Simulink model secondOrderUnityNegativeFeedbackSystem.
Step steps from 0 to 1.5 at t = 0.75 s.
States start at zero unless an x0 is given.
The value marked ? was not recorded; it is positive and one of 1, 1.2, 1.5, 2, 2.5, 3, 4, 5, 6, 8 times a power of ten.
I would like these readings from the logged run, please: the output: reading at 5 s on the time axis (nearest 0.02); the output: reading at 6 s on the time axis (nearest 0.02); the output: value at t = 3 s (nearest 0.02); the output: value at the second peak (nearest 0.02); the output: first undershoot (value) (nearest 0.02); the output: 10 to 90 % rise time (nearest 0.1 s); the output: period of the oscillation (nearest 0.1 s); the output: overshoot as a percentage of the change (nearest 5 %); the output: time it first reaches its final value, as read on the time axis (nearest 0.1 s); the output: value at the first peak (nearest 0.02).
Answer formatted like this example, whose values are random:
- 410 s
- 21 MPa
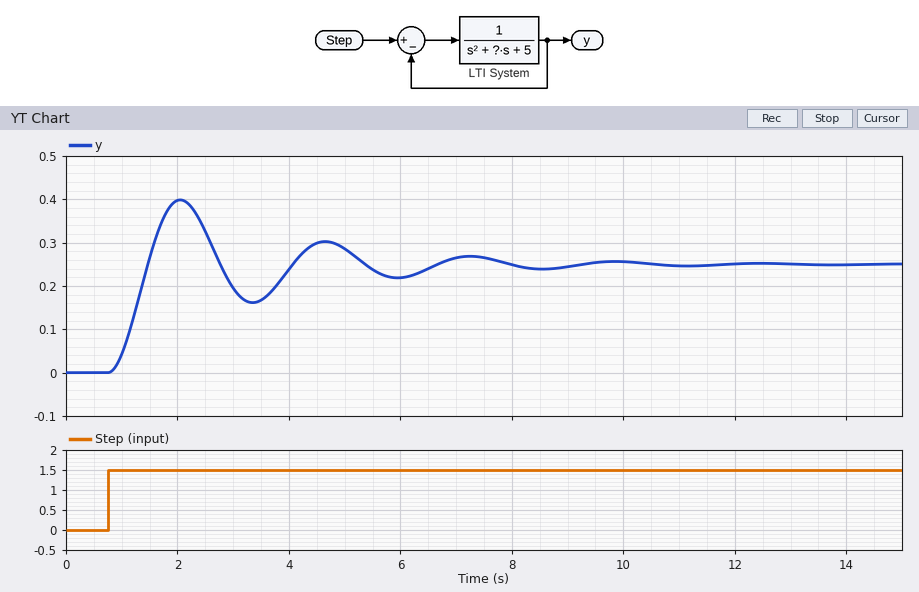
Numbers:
- 0.28
- 0.22
- 0.20
- 0.30
- 0.16
- 0.5 s
- 2.6 s
- 60 %
- 1.5 s
- 0.40
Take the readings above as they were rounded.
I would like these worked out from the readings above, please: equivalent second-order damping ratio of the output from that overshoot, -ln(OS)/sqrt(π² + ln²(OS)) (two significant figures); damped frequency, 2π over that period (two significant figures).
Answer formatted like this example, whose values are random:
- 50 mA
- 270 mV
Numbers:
- 0.16
- 2.4 rad/s
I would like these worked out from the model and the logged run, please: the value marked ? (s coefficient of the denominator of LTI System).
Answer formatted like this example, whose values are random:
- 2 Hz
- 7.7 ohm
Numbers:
- 0.8
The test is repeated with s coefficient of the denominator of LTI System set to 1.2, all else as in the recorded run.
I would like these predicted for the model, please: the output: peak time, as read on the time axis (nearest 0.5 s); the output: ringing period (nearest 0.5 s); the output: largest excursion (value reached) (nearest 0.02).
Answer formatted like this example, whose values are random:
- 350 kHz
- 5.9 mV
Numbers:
- 2.0 s
- 2.5 s
- 0.36
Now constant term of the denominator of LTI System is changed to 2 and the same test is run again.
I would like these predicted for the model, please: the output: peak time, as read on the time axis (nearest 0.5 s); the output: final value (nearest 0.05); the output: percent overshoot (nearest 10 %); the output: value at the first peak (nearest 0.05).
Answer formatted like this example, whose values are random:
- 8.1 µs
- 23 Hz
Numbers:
- 2.5 s
- 0.50
- 50 %
- 0.75
